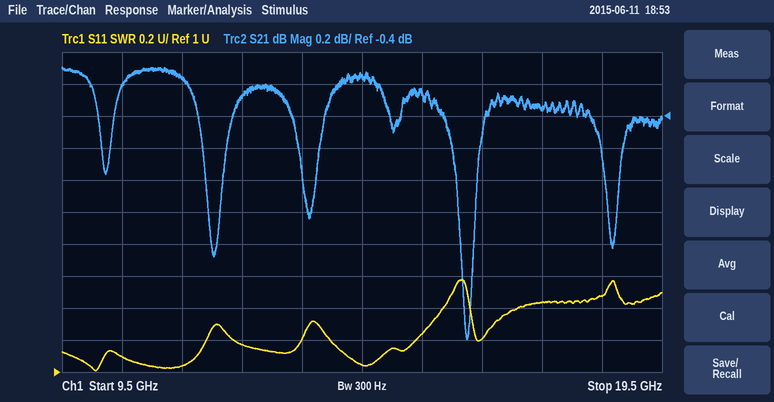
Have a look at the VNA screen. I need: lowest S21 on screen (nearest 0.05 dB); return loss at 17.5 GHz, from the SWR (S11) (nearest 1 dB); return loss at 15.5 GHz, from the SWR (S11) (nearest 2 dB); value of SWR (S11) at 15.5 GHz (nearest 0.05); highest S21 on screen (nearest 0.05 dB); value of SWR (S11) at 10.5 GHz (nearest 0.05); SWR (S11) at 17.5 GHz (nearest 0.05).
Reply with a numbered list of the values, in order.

1. -1.80 dB
2. 15 dB
3. 20 dB
4. 1.25
5. -0.10 dB
6. 1.10
7. 1.45
